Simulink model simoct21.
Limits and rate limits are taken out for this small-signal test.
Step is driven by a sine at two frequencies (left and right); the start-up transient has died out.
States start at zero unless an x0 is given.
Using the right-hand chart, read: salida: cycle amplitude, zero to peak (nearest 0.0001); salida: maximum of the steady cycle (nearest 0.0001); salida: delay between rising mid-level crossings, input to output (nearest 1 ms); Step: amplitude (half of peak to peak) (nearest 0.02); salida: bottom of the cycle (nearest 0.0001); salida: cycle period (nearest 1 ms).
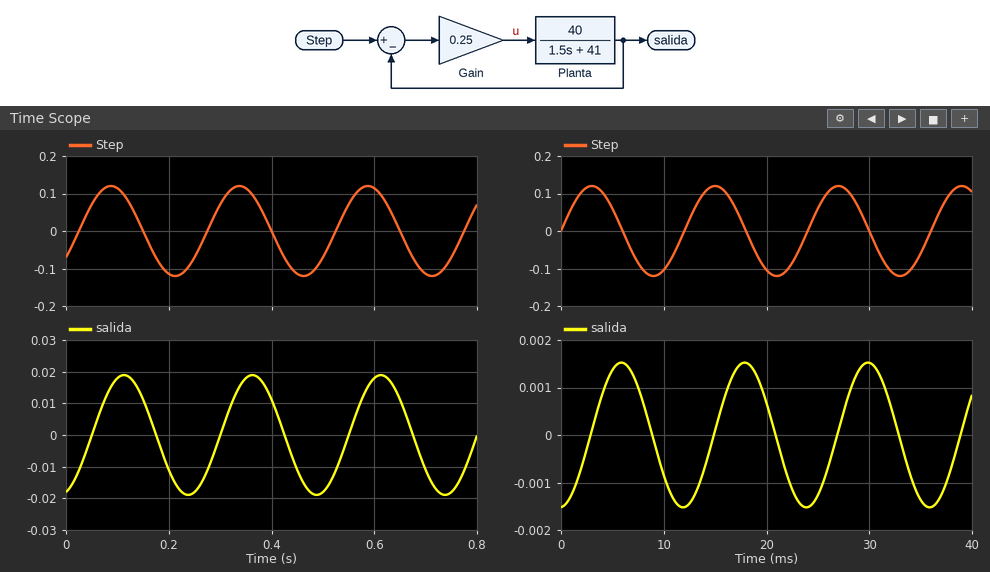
0.0015
0.0015
3 ms
0.12
-0.0015
12 ms
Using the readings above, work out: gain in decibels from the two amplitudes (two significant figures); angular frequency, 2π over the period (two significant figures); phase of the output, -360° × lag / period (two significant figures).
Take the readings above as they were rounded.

-38 dB
0.52 rad/ms
-90°
